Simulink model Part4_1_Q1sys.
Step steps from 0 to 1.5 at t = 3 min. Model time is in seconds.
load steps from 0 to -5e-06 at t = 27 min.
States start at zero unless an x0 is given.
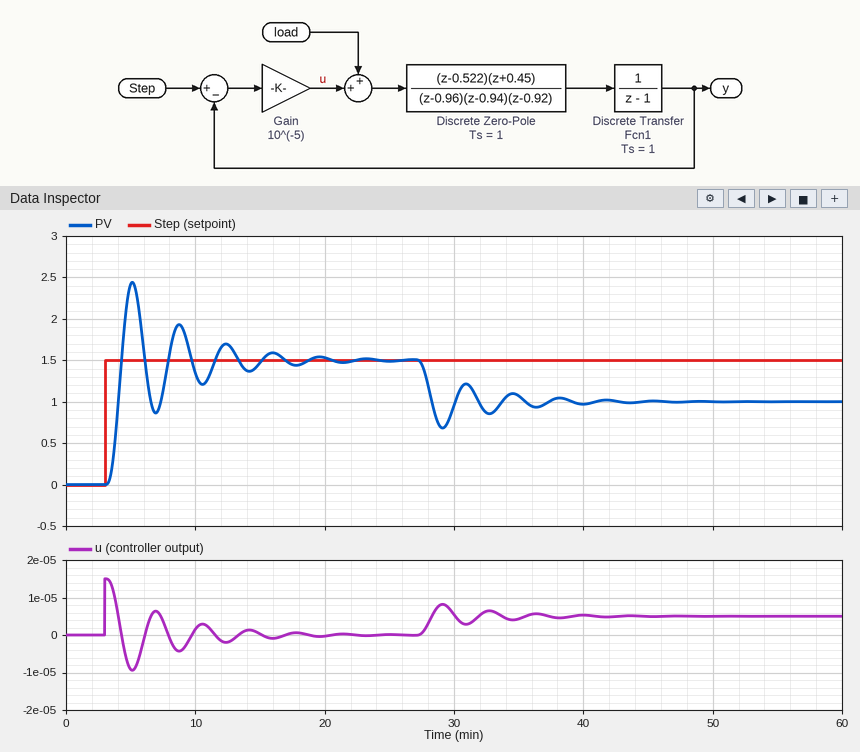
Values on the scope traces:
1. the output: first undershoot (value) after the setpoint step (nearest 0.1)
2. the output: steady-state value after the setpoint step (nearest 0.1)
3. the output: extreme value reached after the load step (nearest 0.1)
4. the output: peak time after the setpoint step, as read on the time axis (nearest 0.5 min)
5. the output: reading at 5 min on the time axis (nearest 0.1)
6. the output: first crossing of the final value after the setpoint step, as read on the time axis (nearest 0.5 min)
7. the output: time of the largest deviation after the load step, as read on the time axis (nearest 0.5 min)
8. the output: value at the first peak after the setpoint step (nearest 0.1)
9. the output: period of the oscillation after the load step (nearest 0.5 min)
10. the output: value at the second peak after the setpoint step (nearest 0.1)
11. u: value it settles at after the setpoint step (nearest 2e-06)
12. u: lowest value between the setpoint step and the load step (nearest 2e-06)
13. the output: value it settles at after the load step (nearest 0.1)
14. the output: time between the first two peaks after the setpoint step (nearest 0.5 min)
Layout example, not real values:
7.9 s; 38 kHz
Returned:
0.9; 1.5; 0.7; 5.0 min; 2.4; 4.5 min; 29.0 min; 2.4; 3.5 min; 1.9; 0.000000; -0.000010; 1.0; 3.5 min
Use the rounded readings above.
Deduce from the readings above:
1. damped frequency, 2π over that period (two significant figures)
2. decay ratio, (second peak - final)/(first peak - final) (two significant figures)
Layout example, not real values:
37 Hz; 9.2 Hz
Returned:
1.8 rad/min; 0.44
